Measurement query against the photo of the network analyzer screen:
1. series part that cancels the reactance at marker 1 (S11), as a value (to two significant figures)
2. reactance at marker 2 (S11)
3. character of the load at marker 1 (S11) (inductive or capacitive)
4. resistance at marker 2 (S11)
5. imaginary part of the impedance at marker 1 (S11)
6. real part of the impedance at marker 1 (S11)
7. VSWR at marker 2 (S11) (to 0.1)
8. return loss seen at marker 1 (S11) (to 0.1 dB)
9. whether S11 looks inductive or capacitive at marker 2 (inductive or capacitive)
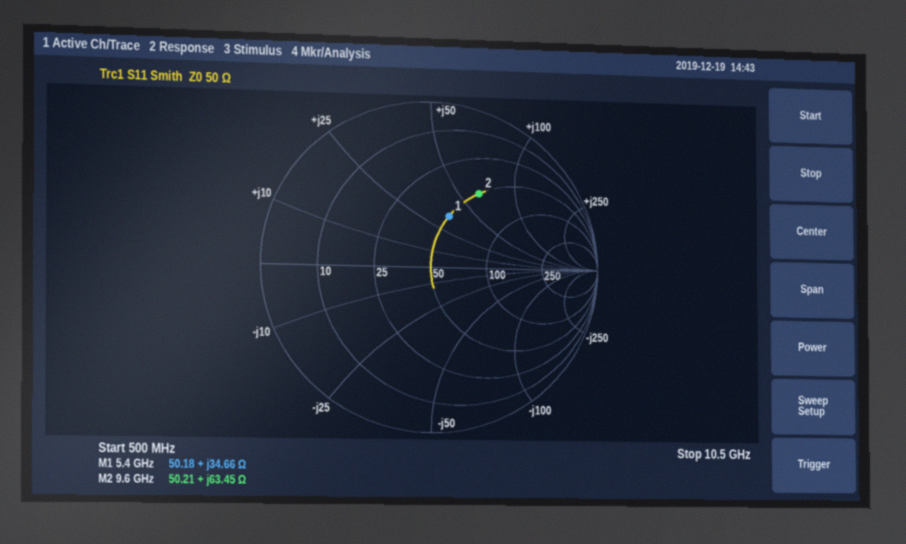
850 fF
+63.45 Ω
inductive
50.21 Ω
+34.66 Ω
50.18 Ω
3.3
9.7 dB
inductive
